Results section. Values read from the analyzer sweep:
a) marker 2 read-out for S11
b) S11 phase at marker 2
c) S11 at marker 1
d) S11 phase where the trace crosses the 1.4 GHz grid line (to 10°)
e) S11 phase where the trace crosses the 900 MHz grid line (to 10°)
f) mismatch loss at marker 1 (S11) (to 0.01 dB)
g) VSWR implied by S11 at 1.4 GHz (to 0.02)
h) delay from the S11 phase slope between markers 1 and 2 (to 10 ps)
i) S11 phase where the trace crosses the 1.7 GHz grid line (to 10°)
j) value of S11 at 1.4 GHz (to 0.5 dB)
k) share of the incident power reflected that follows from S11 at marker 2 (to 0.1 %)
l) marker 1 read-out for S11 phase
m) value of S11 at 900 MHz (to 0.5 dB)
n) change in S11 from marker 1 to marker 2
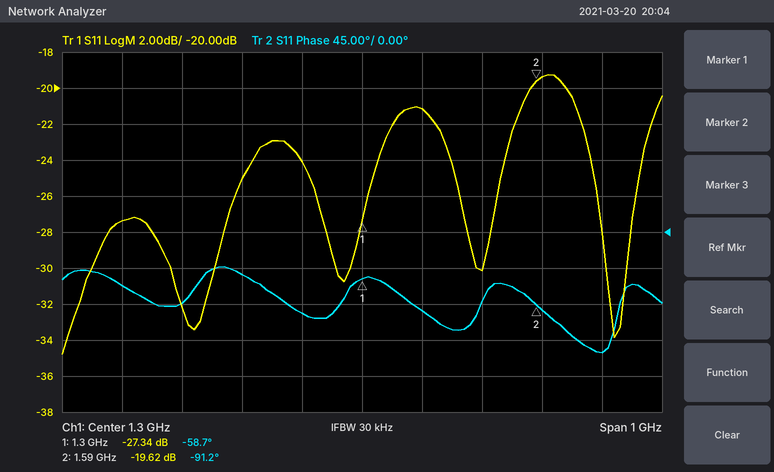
-19.62 dB
-91.2°
-27.34 dB
-100°
-70°
0.01 dB
1.20
310 ps
-150°
-21.0 dB
1.1 %
-58.7°
-27.5 dB
7.72 dB
